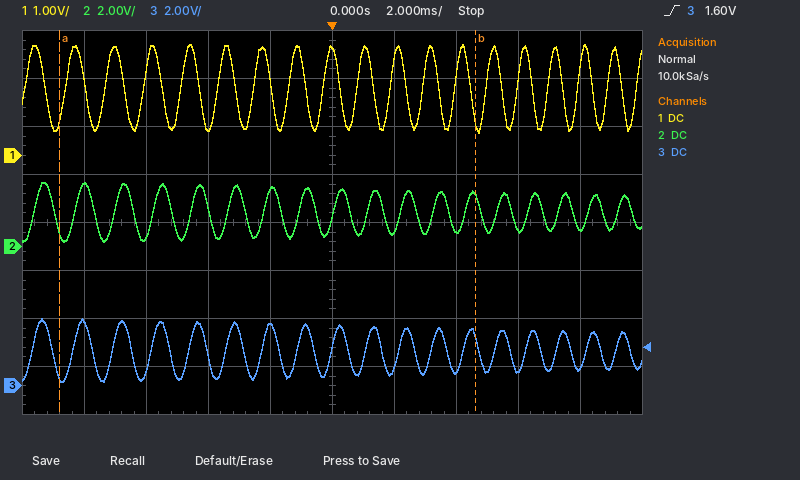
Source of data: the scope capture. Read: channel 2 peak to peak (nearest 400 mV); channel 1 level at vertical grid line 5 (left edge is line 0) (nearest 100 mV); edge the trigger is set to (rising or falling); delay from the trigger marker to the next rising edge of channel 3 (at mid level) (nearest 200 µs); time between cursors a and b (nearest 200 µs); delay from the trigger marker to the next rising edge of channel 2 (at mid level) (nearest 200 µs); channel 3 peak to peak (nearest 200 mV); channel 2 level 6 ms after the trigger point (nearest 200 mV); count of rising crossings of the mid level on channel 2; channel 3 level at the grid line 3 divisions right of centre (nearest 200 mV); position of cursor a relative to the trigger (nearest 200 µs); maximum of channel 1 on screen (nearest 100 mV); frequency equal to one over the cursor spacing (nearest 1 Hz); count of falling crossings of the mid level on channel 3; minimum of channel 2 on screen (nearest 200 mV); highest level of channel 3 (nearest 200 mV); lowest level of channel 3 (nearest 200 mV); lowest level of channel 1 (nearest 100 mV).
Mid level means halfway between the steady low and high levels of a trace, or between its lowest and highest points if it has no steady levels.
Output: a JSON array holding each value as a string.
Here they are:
["2.4 V", "2.2 V", "rising", "1.0 ms", "13.4 ms", "1.2 ms", "2.6 V", "800 mV", "18", "600 mV", "-8.8 ms", "2.3 V", "75 Hz", "18", "200 mV", "2.8 V", "200 mV", "500 mV"]
